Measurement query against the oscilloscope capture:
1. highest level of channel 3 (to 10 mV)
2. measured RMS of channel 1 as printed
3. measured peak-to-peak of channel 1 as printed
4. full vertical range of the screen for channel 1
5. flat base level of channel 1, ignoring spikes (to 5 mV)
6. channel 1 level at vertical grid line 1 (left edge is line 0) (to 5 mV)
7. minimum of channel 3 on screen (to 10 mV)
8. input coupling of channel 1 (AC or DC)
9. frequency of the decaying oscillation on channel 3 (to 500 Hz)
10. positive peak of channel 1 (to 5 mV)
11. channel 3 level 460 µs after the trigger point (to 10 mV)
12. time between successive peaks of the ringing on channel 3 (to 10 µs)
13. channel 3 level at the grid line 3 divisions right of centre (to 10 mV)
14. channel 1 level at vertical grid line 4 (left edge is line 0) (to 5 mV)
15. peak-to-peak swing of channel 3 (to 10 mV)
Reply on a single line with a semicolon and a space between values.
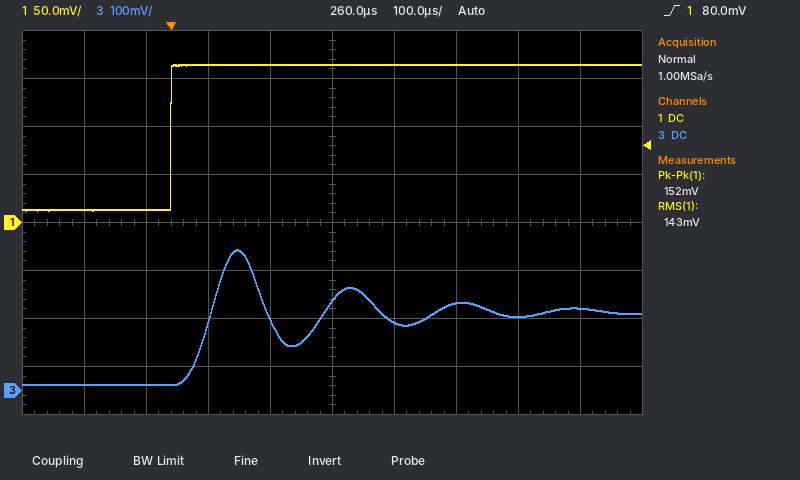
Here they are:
290 mV; 143 mV; 152 mV; 400 mV; 15 mV; 15 mV; 10 mV; DC; 5.5 kHz; 165 mV; 180 mV; 180 µs; 150 mV; 165 mV; 280 mV
